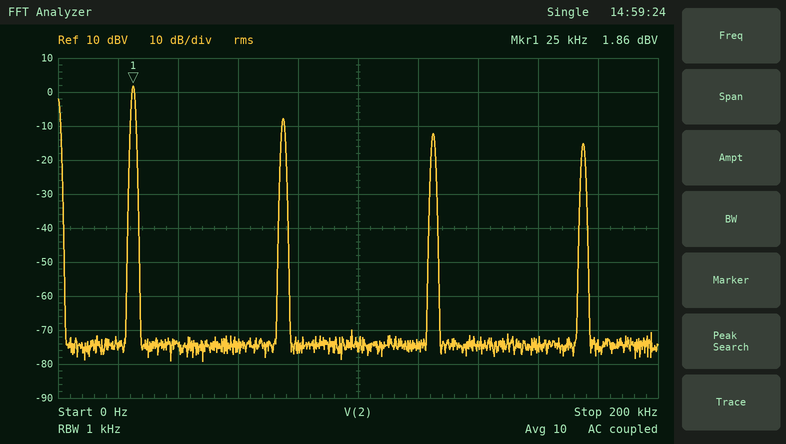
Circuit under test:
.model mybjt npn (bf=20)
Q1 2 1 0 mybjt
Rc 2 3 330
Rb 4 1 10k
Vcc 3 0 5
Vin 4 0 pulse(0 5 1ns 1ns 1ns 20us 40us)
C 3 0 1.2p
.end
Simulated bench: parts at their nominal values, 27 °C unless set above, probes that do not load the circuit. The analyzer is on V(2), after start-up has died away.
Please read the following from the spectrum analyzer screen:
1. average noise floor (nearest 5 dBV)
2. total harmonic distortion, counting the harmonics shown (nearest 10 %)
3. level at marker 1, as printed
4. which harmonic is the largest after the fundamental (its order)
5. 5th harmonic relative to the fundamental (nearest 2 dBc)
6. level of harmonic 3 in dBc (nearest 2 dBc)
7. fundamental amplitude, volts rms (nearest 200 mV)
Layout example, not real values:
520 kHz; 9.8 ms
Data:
-75 dBV; 40 %; 1.86 dBV; 3; -14 dBc; -10 dBc; 1.2 V
